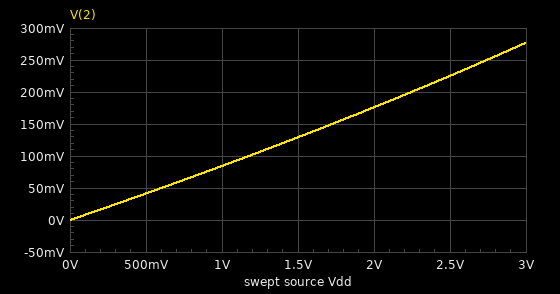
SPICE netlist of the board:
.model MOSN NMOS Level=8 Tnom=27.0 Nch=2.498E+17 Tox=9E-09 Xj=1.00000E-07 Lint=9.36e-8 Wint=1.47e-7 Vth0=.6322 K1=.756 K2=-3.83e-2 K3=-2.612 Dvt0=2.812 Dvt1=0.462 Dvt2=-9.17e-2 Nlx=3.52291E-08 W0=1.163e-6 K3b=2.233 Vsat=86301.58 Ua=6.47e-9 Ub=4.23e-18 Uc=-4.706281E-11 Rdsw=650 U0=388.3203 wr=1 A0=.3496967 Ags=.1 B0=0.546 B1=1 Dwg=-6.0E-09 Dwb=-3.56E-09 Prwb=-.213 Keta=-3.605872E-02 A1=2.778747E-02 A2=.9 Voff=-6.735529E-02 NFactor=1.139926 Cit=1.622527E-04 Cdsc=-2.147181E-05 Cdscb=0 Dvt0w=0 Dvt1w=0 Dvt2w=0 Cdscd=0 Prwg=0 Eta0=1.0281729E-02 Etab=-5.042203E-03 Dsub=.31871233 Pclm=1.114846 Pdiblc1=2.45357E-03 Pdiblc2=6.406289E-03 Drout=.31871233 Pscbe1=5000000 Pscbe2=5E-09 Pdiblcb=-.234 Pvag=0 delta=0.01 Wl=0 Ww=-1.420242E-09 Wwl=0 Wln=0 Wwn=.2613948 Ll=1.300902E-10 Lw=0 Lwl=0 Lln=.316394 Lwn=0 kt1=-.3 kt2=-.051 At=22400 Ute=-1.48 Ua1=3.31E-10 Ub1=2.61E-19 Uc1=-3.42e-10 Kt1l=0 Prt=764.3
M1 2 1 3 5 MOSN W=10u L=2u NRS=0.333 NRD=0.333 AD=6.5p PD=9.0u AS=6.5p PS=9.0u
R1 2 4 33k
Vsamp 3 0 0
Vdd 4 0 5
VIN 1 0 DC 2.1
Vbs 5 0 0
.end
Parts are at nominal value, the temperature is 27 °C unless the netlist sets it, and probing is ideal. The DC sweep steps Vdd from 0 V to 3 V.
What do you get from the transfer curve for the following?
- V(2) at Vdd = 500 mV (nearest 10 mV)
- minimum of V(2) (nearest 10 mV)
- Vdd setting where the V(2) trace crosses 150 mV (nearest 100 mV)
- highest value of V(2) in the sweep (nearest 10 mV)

40 mV
0 V
1.7 V
280 mV
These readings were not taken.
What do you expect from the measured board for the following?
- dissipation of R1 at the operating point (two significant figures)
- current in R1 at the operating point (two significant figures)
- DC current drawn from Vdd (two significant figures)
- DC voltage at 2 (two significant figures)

610 µW
140 µA
140 µA
520 mV
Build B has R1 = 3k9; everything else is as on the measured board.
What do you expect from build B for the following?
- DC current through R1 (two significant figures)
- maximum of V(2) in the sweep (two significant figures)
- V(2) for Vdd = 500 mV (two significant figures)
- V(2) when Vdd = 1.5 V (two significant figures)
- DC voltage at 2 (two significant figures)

200 µA
2.2 V
230 mV
820 mV
4.2 V
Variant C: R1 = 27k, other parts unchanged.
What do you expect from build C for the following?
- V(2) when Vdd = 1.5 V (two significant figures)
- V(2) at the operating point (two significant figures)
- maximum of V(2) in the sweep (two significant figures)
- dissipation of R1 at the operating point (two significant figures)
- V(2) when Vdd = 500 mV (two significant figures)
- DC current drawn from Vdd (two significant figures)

160 mV
680 mV
340 mV
690 µW
50 mV
160 µA
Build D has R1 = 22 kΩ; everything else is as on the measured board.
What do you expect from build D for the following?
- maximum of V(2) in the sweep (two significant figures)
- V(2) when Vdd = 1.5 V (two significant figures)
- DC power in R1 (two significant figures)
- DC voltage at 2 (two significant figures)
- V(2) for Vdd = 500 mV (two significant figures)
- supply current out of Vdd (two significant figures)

430 mV
190 mV
740 µW
960 mV
60 mV
180 µA
